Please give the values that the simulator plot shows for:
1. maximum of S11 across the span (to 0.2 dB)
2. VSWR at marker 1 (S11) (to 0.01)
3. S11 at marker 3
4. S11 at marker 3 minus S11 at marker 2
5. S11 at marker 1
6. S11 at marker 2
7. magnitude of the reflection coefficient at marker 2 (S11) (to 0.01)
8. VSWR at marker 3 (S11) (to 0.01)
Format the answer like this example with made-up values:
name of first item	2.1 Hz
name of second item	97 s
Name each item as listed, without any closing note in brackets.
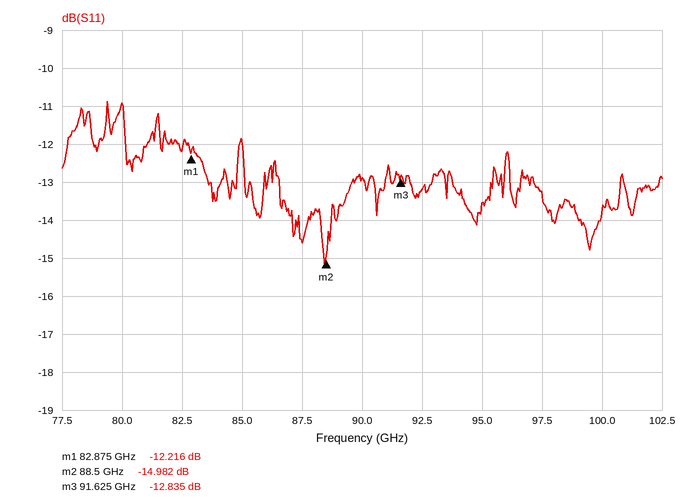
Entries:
maximum of S11 across the span	-10.8 dB
VSWR at marker 1 (S11)	1.65
S11 at marker 3	-12.835 dB
S11 at marker 3 minus S11 at marker 2	2.147 dB
S11 at marker 1	-12.216 dB
S11 at marker 2	-14.982 dB
magnitude of the reflection coefficient at marker 2 (S11)	0.18
VSWR at marker 3 (S11)	1.59
